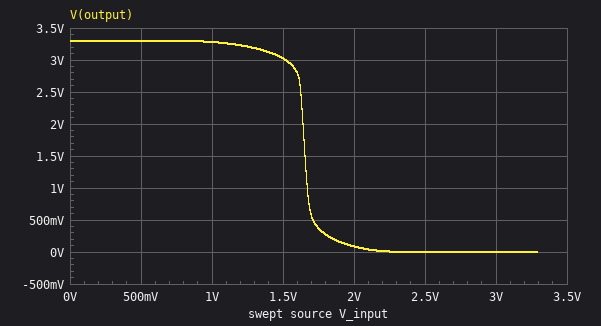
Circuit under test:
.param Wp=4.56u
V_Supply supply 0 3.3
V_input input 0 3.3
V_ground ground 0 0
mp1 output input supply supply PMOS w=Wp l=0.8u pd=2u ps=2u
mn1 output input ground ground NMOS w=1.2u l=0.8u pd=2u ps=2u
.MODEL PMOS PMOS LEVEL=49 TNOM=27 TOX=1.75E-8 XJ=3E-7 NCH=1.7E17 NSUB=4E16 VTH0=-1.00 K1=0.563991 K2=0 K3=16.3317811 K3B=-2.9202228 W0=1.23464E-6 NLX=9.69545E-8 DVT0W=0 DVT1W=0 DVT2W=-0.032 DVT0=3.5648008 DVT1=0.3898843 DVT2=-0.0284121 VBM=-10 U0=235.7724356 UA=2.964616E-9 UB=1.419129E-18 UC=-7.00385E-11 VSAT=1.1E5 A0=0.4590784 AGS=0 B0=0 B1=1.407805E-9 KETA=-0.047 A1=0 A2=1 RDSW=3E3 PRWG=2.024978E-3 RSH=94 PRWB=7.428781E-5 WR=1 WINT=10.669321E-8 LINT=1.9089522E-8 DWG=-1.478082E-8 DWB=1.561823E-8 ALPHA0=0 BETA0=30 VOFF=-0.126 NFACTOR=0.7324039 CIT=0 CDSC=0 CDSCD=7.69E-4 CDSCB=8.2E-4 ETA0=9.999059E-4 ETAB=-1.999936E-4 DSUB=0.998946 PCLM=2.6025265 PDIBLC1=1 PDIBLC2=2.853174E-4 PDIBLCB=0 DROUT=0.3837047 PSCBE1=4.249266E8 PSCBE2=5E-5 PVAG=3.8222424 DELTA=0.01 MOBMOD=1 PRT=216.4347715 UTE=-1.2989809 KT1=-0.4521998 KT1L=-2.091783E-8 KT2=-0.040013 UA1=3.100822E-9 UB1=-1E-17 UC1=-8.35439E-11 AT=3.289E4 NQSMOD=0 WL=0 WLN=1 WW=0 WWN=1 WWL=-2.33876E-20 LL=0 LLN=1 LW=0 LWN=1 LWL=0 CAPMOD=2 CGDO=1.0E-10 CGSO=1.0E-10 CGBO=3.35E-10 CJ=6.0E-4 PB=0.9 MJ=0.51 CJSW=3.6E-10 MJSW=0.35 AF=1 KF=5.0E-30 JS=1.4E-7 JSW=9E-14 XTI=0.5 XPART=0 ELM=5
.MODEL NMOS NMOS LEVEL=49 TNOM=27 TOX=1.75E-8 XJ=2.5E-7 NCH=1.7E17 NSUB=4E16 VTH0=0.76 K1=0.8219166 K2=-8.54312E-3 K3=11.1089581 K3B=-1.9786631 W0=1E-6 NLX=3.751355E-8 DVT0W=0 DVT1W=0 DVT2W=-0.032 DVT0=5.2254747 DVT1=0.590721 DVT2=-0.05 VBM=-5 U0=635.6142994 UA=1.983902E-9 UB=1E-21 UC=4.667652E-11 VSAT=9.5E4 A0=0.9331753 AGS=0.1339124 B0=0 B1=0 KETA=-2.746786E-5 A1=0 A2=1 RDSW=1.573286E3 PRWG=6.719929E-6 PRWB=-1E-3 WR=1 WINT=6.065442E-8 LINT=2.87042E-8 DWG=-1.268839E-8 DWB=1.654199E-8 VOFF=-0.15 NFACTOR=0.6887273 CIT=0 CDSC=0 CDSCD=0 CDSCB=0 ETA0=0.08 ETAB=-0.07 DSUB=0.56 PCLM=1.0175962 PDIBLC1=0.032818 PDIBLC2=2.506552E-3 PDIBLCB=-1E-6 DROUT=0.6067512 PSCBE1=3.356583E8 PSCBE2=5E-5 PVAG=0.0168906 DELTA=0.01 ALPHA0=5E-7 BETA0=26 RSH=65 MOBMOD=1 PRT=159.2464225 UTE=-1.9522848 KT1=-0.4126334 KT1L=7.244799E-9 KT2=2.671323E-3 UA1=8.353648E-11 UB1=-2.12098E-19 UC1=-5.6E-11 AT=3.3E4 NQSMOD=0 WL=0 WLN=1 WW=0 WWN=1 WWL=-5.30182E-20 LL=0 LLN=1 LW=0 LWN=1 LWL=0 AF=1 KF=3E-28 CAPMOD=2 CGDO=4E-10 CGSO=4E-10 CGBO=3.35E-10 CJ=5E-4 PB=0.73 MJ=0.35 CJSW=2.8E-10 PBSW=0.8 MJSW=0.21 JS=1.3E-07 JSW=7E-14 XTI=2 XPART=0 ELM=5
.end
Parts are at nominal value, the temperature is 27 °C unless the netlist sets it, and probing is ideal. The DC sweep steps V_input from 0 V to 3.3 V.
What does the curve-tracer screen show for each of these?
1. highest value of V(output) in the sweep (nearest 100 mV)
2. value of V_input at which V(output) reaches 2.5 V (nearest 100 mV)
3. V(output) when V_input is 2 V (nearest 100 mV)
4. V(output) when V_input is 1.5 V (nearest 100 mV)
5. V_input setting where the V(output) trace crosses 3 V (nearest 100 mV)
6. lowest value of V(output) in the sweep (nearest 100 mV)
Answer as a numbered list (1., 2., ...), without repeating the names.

1. 3.3 V
2. 1.6 V
3. 100 mV
4. 3.0 V
5. 1.5 V
6. 0 V
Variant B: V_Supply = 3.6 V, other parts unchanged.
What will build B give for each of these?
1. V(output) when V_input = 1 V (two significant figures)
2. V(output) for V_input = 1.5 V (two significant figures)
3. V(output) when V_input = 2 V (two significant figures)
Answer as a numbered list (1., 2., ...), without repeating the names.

1. 3.6 V
2. 3.4 V
3. 330 mV
